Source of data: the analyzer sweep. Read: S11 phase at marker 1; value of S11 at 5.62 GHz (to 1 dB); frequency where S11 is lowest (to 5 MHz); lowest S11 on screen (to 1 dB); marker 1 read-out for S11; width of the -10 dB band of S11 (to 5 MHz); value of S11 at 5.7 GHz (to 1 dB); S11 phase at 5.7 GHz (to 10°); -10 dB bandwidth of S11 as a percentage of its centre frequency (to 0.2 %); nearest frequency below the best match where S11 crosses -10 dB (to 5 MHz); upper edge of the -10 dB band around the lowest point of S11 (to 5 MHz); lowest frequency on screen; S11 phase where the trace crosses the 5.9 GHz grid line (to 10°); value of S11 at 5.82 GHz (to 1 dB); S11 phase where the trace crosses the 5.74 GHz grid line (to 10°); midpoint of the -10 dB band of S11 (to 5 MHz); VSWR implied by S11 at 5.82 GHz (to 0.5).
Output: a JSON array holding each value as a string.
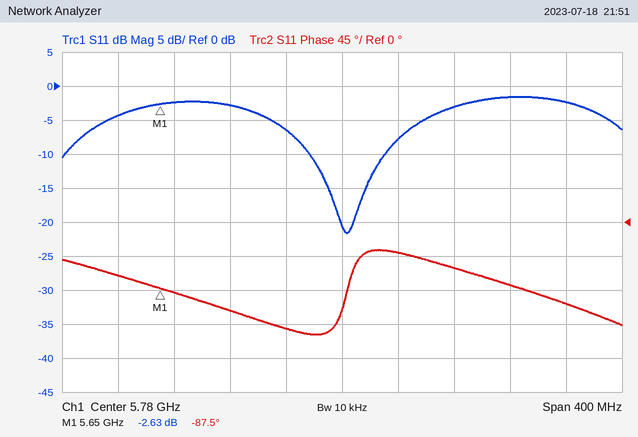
["-87.5°", "-4 dB", "5.785 GHz", "-22 dB", "-2.63 dB", "55 MHz", "-3 dB", "-120°", "1.0 %", "5.755 GHz", "5.810 GHz", "5.58 GHz", "-80°", "-8 dB", "-140°", "5.785 GHz", "2.5"]
